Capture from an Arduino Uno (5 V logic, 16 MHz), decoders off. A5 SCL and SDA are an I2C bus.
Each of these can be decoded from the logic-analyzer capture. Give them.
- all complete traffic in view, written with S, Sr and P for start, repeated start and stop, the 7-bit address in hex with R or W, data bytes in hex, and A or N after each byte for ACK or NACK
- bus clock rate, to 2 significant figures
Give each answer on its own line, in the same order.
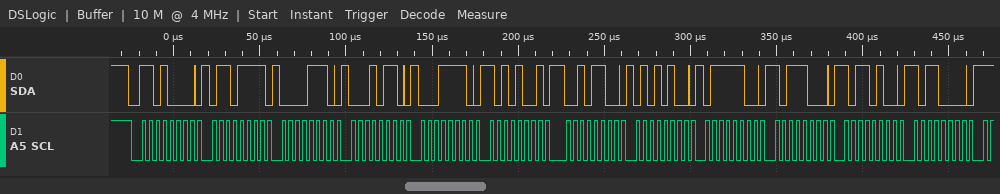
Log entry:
S 68W A 6F A 0E A 16 A 1E A A9 A 2C A 54 A 7C A B8 A B4 A B0 A
250 kHz
